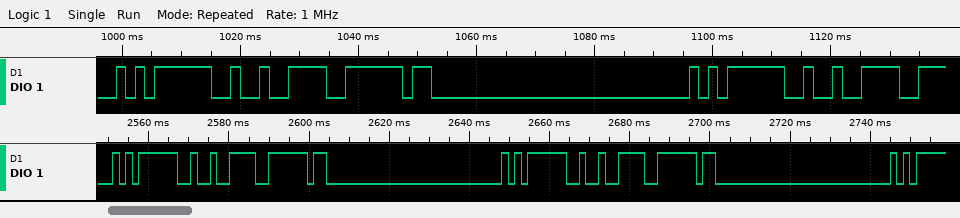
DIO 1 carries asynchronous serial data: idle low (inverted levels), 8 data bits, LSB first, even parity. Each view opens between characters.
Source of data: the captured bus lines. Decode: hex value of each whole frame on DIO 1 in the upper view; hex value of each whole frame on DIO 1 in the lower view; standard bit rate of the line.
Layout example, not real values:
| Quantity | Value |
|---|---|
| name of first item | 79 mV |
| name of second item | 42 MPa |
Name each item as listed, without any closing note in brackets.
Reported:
| Quantity | Value |
|---|---|
| hex value of each whole frame on DIO 1 in the upper view | 05, 1B, 20, 05, 1B |
| hex value of each whole frame on DIO 1 in the lower view | 05, 1B, 20, 05, 1B, 20 |
| standard bit rate of the line | 600 baud |
